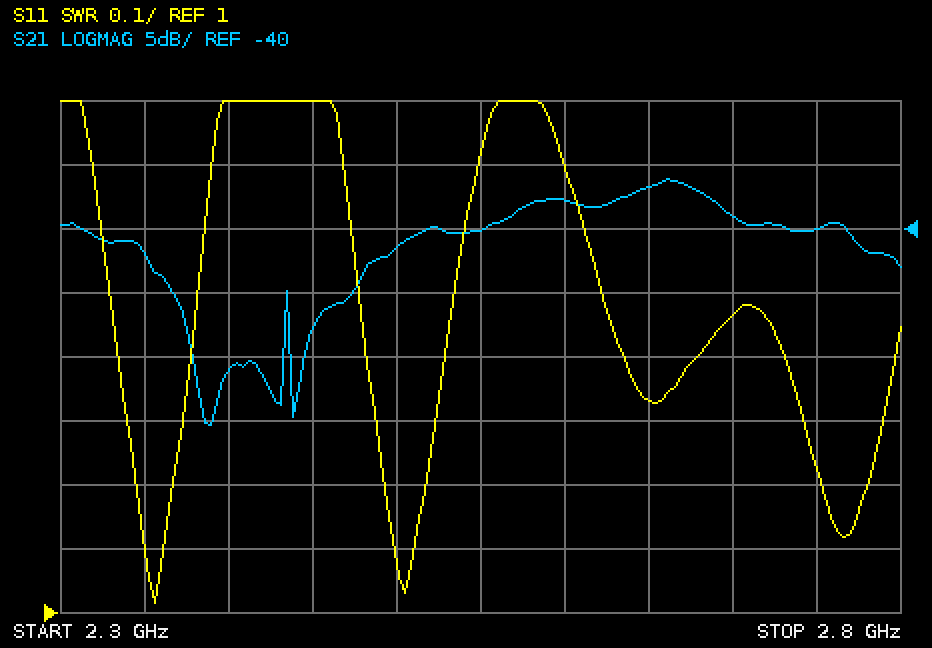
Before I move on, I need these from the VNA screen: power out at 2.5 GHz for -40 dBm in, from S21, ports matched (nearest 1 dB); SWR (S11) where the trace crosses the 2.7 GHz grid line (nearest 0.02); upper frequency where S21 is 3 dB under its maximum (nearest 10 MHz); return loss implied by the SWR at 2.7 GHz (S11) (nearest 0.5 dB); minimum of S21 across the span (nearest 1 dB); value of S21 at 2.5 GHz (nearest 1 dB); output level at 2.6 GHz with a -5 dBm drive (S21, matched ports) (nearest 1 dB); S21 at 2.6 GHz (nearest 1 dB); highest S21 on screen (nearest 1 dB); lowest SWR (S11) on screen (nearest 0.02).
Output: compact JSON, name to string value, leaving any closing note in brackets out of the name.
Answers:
{"power out at 2.5 GHz for -40 dBm in, from S21, ports matched": "-81 dBm", "SWR (S11) where the trace crosses the 2.7 GHz grid line": "1.46", "upper frequency where S21 is 3 dB under its maximum": "2.70 GHz", "return loss implied by the SWR at 2.7 GHz (S11)": "14.5 dB", "minimum of S21 across the span": "-55 dB", "value of S21 at 2.5 GHz": "-41 dB", "output level at 2.6 GHz with a -5 dBm drive (S21, matched ports)": "-43 dBm", "S21 at 2.6 GHz": "-38 dB", "highest S21 on screen": "-36 dB", "lowest SWR (S11) on screen": "1.02"}
